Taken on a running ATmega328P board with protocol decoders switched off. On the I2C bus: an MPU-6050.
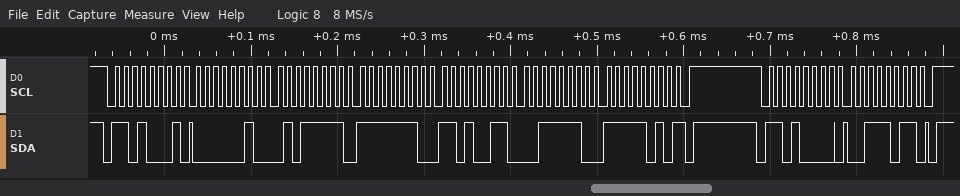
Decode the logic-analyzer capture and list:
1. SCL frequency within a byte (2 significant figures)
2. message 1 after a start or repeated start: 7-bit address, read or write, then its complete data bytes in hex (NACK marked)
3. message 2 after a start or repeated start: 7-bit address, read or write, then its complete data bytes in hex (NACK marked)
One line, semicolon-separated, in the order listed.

100 kHz; 0x68 read: 02 5F FE D3 3E FA NACK; 0x68 write: 3B
